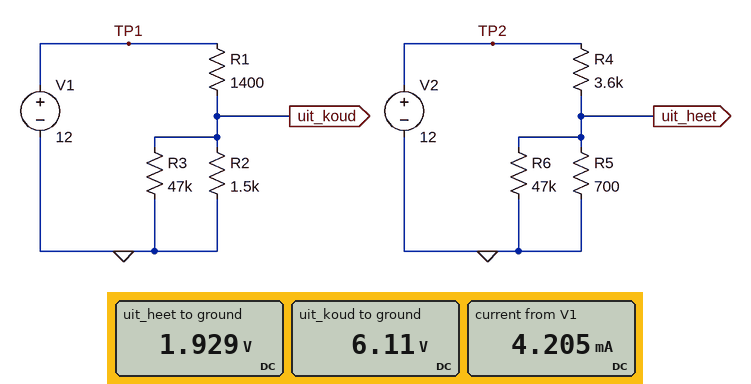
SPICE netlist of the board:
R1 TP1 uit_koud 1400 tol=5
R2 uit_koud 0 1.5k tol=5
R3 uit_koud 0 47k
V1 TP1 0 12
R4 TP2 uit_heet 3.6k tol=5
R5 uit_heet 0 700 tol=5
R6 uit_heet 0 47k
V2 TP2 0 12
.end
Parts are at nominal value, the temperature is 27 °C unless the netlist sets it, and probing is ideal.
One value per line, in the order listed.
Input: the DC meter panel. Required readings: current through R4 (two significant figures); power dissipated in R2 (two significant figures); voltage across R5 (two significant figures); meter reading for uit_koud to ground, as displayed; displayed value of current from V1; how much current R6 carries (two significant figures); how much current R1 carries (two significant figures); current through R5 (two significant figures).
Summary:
2.8 mA
25 mW
1.9 V
6.11 V
4.205 mA
41 µA
4.2 mA
2.8 mA
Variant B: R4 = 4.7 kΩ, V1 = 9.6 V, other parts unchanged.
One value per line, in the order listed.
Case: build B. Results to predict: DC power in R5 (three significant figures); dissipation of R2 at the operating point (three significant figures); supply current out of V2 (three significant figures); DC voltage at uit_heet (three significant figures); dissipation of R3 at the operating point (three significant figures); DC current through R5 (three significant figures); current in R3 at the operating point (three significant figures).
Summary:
3.37 mW
15.9 mW
2.23 mA
1.54 V
509 µW
2.19 mA
104 µA
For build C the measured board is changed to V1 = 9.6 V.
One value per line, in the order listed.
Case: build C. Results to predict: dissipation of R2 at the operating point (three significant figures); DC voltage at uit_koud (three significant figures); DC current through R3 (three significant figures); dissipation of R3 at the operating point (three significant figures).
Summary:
15.9 mW
4.89 V
104 µA
509 µW
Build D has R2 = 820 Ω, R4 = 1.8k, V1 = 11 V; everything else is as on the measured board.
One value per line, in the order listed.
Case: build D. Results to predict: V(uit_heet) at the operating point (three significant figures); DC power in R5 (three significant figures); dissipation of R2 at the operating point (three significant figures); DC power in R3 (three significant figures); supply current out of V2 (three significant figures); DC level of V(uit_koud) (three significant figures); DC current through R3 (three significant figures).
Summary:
3.32 V
15.8 mW
19.7 mW
344 µW
4.82 mA
4.02 V
85.5 µA
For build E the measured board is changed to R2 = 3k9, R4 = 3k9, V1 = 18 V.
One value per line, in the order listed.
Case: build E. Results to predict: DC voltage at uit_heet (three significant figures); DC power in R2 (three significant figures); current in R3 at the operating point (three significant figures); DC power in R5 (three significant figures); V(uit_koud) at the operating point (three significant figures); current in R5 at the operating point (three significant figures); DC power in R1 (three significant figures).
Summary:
1.80 V
43.1 mW
276 µA
4.65 mW
13.0 V
2.58 mA
18.1 mW
